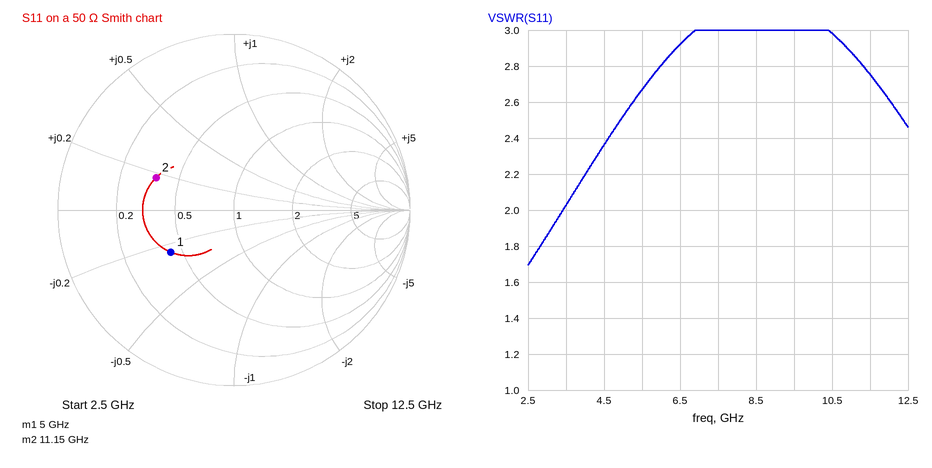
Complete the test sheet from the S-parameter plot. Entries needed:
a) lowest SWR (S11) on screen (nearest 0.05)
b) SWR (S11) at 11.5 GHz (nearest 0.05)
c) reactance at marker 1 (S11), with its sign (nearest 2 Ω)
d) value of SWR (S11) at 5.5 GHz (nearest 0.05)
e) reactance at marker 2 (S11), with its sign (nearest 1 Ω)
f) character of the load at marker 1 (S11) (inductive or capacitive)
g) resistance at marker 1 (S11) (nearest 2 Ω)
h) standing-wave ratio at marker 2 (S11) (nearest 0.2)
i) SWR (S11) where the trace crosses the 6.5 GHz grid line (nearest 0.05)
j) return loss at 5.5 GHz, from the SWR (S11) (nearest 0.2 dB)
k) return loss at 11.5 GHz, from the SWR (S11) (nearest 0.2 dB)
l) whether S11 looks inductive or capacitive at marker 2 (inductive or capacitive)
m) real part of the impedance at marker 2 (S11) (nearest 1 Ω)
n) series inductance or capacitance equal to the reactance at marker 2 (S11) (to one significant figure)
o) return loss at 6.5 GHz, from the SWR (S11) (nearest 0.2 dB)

1.70
2.75
-12 Ω
2.65
+9 Ω
capacitive
22 Ω
2.8
2.90
6.8 dB
6.6 dB
inductive
18 Ω
100 pH
6.2 dB
